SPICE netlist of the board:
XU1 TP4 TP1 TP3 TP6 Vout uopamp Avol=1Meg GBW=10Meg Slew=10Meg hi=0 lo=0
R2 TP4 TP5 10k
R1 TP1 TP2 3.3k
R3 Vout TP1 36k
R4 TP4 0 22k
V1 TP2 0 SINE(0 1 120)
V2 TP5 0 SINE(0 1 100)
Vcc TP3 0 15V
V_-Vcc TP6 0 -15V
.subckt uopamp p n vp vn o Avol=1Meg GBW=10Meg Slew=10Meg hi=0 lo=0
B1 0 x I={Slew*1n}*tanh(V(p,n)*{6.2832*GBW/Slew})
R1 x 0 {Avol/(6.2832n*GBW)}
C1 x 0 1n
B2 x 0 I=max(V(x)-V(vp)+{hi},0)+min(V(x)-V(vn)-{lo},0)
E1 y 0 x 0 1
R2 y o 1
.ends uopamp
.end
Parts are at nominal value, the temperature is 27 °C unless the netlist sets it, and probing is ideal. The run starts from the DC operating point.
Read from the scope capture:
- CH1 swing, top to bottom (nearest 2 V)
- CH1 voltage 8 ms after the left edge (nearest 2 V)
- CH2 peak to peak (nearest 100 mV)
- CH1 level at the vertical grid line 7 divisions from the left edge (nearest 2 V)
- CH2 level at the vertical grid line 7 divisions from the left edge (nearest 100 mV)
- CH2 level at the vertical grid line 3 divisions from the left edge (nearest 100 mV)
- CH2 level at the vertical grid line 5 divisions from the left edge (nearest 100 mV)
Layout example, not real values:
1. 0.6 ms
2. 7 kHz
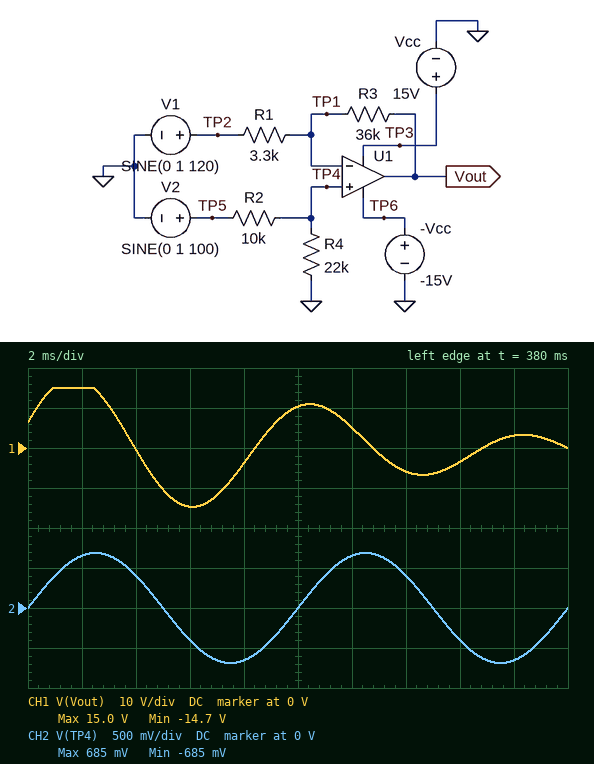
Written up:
1. 30 V
2. -4 V
3. 1.4 V
4. -6 V
5. 400 mV
6. -400 mV
7. 0 V
